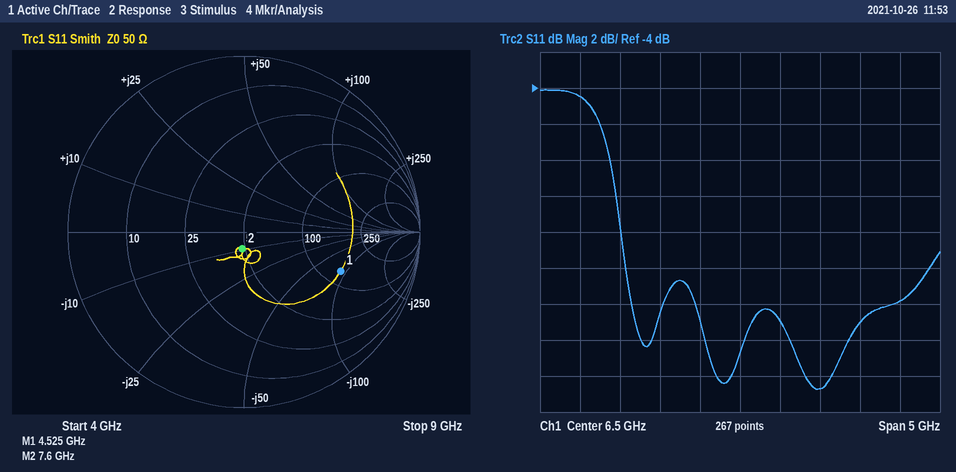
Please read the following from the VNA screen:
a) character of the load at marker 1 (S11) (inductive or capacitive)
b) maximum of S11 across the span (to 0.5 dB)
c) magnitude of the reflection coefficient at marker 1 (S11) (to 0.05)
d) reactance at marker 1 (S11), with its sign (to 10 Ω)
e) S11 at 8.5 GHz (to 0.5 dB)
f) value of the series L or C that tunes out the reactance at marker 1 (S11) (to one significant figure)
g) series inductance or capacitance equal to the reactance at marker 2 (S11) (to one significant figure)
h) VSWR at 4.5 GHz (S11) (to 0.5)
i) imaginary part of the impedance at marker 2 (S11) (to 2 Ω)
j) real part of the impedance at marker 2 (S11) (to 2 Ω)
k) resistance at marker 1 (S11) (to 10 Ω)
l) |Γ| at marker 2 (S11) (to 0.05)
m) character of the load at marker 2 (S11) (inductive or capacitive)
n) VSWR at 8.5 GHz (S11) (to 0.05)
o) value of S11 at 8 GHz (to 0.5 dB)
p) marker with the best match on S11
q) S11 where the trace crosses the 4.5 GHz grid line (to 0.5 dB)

capacitive
-4.0 dB
0.60
-90 Ω
-16.0 dB
3 nH
2 pF
4.0
-10 Ω
48 Ω
130 Ω
0.10
capacitive
1.40
-17.0 dB
marker 2
-4.5 dB
